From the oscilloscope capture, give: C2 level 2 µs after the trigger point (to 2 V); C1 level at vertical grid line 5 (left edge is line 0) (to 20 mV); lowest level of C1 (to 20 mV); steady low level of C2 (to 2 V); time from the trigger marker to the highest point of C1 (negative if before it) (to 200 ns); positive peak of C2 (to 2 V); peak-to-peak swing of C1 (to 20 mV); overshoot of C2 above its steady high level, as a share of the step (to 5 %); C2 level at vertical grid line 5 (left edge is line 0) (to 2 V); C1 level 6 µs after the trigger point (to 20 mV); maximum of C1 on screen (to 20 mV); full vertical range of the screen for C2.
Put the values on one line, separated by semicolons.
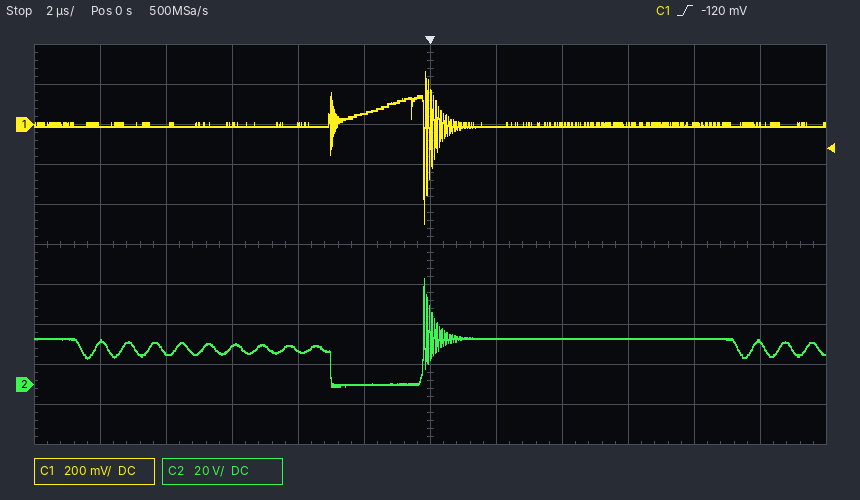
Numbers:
24 V; 60 mV; -500 mV; 0 V; -200 ns; 52 V; 760 mV; 130 %; 0 V; 0 mV; 260 mV; 200 V
